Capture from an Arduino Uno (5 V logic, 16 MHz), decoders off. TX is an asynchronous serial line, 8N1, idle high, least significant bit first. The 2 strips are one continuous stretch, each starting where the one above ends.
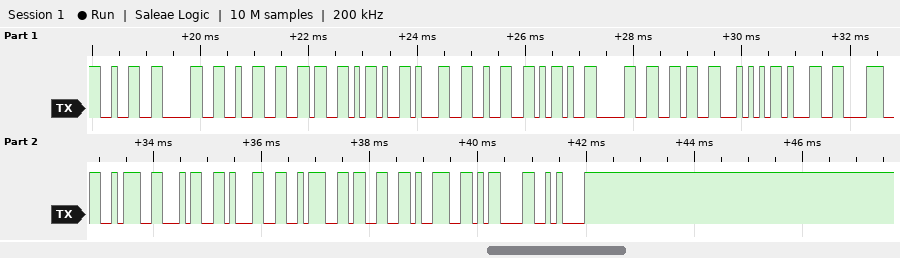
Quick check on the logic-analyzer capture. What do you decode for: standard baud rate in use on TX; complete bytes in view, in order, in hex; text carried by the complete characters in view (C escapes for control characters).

9600 baud
32 30 32 36 2D 31 32 2D 30 36 54 31 38 3A 34 31 3A 33 39 0D 0A
"2026-12-06T18:41:39\r\n"
